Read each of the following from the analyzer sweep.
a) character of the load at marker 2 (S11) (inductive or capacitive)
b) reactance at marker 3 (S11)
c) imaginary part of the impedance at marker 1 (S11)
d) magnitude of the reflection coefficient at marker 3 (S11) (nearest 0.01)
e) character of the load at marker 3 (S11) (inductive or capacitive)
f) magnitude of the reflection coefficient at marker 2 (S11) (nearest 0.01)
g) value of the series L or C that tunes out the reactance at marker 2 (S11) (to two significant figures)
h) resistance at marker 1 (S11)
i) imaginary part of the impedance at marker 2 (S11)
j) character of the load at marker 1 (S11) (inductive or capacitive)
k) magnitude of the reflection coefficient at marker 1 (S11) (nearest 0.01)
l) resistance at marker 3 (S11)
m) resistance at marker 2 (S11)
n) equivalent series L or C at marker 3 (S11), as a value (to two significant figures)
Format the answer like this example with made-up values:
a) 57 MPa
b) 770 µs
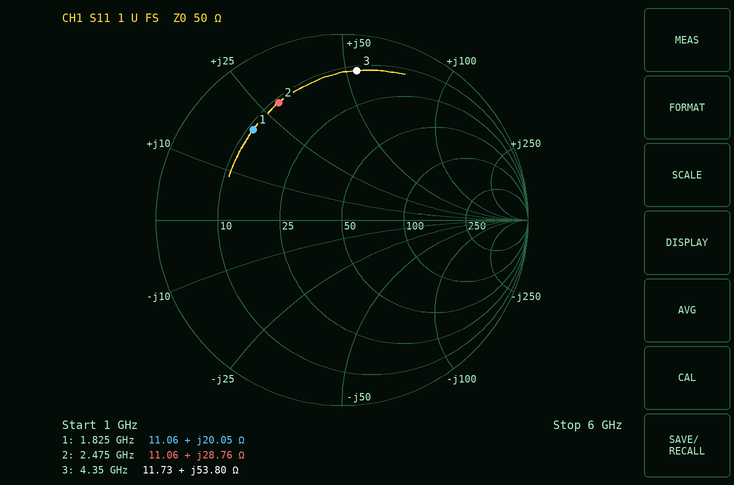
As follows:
a) inductive
b) +53.80 Ω
c) +20.05 Ω
d) 0.81
e) inductive
f) 0.72
g) 2.2 pF
h) 11.06 Ω
i) +28.76 Ω
j) inductive
k) 0.68
l) 11.73 Ω
m) 11.06 Ω
n) 2.0 nH
